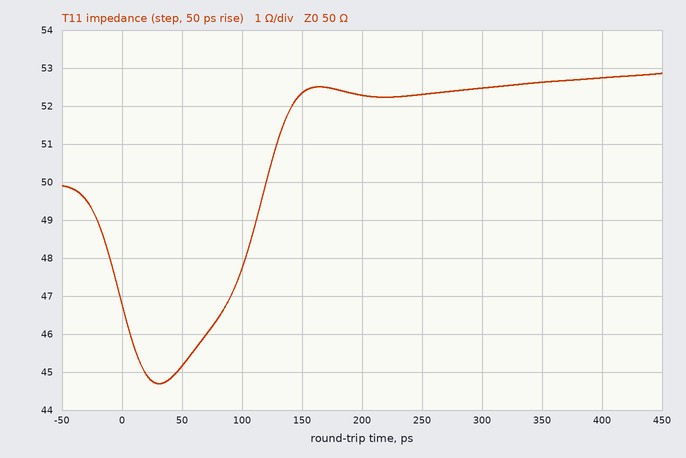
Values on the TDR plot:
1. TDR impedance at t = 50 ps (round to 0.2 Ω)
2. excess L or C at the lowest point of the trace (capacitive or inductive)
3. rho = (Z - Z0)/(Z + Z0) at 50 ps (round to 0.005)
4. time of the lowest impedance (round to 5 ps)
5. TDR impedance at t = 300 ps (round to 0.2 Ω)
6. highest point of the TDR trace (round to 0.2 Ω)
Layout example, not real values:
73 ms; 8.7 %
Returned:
45.2 Ω; capacitive; -0.050; 30 ps; 52.4 Ω; 52.8 Ω
